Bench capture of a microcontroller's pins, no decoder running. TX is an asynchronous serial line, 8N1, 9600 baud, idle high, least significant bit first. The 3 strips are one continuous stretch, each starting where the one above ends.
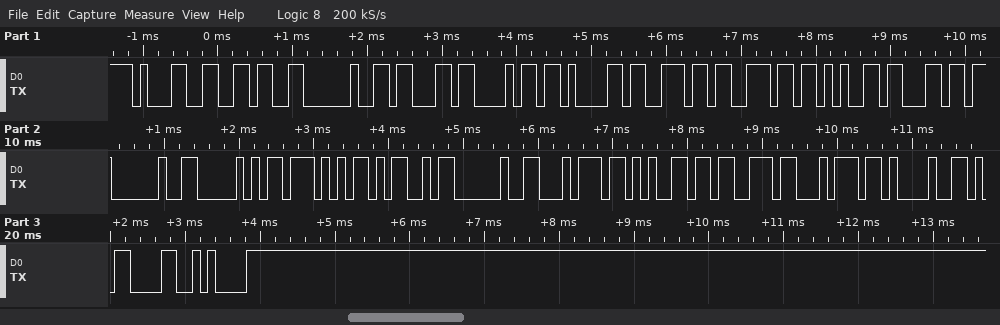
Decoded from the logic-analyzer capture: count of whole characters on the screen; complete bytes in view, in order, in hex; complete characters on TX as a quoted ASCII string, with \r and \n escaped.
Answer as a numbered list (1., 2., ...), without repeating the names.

1. 22
2. 31 36 20 63 68 61 6E 6E 65 6C 20 50 57 4D 20 74 65 73 74 21 0D 0A
3. "16 channel PWM test!\r\n"
